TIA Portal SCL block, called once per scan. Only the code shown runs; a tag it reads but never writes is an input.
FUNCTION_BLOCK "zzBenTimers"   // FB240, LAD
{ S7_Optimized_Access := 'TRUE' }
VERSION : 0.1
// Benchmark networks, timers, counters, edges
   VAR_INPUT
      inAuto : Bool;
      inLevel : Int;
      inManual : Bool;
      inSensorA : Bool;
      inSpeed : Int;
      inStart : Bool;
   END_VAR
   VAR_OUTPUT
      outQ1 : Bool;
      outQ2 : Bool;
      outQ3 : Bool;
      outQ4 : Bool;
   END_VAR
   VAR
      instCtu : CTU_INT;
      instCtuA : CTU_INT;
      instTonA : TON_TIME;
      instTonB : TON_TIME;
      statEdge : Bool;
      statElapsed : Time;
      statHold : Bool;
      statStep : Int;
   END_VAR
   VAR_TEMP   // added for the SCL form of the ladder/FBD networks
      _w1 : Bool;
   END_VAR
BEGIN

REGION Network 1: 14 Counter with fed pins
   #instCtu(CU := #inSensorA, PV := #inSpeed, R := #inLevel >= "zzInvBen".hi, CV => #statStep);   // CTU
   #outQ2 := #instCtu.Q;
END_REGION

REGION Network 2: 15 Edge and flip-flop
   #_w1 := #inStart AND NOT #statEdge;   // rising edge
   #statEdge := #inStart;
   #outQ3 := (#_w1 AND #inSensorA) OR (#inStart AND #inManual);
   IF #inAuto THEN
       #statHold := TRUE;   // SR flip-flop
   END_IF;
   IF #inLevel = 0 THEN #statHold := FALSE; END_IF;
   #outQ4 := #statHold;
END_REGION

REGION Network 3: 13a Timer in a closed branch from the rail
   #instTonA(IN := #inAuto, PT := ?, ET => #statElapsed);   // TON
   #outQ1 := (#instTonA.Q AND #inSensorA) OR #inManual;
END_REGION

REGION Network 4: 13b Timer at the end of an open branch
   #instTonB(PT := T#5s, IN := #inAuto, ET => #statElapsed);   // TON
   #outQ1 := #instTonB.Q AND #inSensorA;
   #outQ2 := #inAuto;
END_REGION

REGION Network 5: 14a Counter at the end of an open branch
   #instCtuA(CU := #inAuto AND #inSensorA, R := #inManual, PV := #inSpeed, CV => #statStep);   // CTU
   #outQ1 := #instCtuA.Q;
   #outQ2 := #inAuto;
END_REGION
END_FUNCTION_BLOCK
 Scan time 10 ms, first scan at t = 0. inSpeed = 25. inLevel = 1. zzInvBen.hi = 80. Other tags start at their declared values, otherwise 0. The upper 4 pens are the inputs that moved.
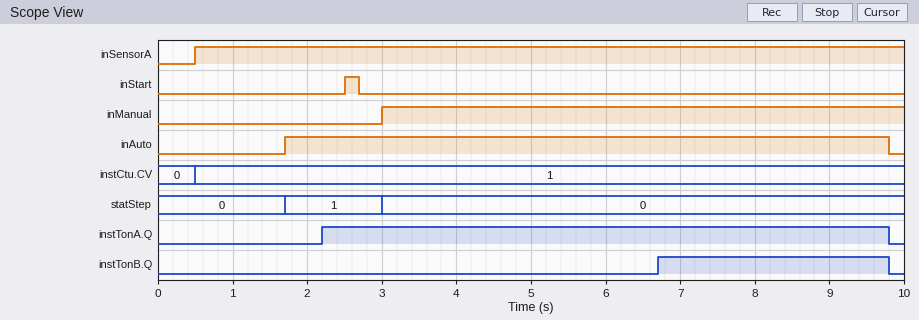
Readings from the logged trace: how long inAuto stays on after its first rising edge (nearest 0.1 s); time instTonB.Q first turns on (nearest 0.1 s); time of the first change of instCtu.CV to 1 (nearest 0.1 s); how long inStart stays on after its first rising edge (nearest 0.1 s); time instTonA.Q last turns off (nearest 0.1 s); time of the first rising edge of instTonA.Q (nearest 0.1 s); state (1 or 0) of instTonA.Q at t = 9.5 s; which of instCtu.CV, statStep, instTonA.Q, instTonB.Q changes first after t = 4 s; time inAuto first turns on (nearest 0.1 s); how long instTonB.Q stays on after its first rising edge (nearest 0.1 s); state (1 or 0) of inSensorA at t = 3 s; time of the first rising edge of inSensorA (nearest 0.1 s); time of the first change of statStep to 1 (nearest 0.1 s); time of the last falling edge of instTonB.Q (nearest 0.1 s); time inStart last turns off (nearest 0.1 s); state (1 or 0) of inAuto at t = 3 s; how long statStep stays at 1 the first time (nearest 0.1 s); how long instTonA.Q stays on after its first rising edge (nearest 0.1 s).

8.1 s
6.7 s
0.5 s
0.2 s
9.8 s
2.2 s
1
instTonB.Q
1.7 s
3.1 s
1
0.5 s
1.7 s
9.8 s
2.7 s
1
1.3 s
7.6 s
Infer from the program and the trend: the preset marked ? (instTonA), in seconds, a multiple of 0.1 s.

0.5 s
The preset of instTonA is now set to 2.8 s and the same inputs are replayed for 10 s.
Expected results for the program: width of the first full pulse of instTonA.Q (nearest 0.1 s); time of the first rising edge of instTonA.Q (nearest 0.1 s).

5.3 s
4.5 s
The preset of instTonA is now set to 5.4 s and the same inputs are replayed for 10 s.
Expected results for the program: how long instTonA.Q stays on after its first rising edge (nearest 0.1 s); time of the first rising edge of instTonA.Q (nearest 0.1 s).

2.7 s
7.1 s
